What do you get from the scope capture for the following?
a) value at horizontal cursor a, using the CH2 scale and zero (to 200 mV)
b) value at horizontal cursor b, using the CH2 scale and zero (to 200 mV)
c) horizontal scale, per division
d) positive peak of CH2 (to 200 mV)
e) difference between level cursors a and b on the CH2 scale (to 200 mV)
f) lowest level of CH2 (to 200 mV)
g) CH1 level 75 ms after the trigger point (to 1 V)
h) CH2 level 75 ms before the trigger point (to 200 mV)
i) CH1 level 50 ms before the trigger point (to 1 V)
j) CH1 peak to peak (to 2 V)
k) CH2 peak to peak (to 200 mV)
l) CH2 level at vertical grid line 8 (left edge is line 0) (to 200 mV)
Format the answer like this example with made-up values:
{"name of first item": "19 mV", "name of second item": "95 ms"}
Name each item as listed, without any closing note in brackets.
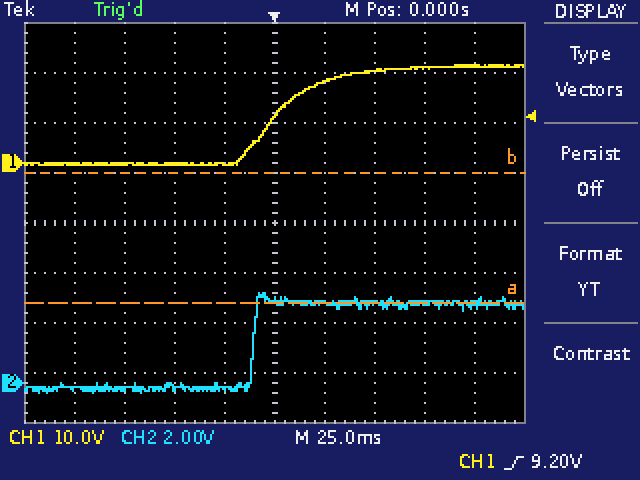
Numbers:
{"value at horizontal cursor a, using the CH2 scale and zero": "3.2 V", "value at horizontal cursor b, using the CH2 scale and zero": "8.4 V", "horizontal scale, per division": "25 ms", "positive peak of CH2": "3.6 V", "difference between level cursors a and b on the CH2 scale": "5.2 V", "lowest level of CH2": "-400 mV", "CH1 level 75 ms after the trigger point": "19 V", "CH2 level 75 ms before the trigger point": "-200 mV", "CH1 level 50 ms before the trigger point": "0 V", "CH1 peak to peak": "20 V", "CH2 peak to peak": "4.0 V", "CH2 level at vertical grid line 8 (left edge is line 0)": "3.2 V"}
